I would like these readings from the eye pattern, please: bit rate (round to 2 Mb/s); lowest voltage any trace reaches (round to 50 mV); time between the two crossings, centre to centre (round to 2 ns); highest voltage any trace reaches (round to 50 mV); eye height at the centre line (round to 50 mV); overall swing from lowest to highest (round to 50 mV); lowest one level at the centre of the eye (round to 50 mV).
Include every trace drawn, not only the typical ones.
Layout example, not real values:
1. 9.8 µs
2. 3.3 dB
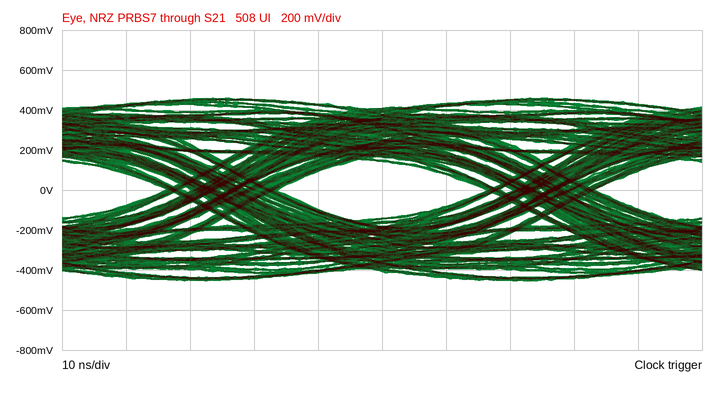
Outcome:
1. 20 Mb/s
2. -450 mV
3. 50 ns
4. 450 mV
5. 300 mV
6. 900 mV
7. 150 mV
